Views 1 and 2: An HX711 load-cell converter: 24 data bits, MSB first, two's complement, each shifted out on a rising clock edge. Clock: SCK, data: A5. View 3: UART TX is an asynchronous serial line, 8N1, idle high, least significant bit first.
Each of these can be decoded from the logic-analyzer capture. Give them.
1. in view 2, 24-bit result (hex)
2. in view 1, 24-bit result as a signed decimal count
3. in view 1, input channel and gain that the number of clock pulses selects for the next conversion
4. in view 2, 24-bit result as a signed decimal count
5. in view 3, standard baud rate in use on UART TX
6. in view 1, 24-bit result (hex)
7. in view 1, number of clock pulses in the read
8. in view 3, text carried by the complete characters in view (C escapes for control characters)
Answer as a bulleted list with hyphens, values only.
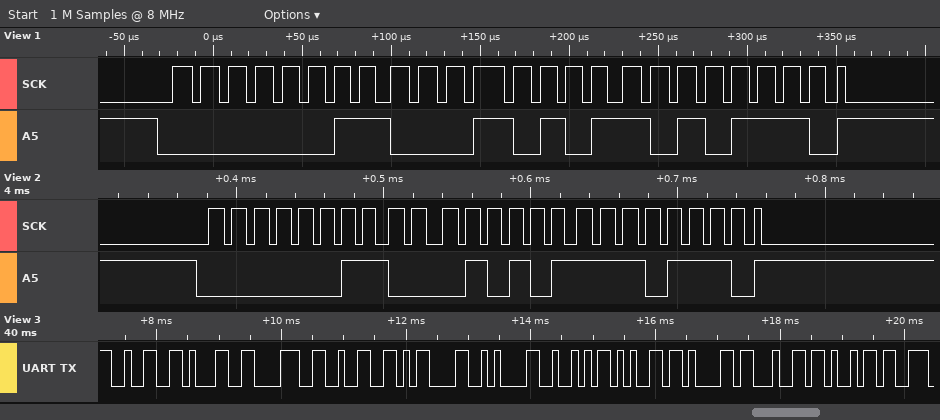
- 0x0315EE
- 202158
- channel A, gain 128
- 202222
- 9600 baud
- 0x0315AE
- 25
- "2182\r\nReadi"
